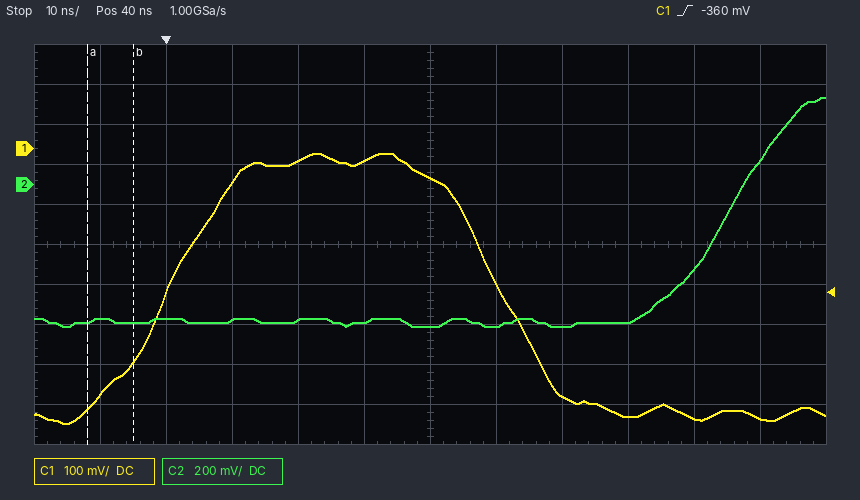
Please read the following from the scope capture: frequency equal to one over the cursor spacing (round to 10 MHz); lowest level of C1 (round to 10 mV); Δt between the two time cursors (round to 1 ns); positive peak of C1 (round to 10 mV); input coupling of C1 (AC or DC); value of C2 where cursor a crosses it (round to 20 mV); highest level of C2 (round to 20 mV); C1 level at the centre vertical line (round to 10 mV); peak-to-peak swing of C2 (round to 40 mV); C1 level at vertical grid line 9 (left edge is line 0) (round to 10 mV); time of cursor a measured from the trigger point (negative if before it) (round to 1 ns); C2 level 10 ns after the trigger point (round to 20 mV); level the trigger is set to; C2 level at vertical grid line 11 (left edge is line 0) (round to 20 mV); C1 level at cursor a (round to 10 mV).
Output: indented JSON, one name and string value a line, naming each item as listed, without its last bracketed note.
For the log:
{
  "frequency equal to one over the cursor spacing": "140 MHz",
  "lowest level of C1": "-690 mV",
  "Δt between the two time cursors": "7 ns",
  "positive peak of C1": "-10 mV",
  "input coupling of C1": "DC",
  "value of C2 where cursor a crosses it": "-680 mV",
  "highest level of C2": "440 mV",
  "C1 level at the centre vertical line": "-70 mV",
  "peak-to-peak swing of C2": "1.16 V",
  "C1 level at vertical grid line 9 (left edge is line 0)": "-670 mV",
  "time of cursor a measured from the trigger point (negative if before it)": "-12 ns",
  "C2 level 10 ns after the trigger point": "-680 mV",
  "level the trigger is set to": "-360 mV",
  "C2 level at vertical grid line 11 (left edge is line 0)": "120 mV",
  "C1 level at cursor a": "-650 mV"
}
